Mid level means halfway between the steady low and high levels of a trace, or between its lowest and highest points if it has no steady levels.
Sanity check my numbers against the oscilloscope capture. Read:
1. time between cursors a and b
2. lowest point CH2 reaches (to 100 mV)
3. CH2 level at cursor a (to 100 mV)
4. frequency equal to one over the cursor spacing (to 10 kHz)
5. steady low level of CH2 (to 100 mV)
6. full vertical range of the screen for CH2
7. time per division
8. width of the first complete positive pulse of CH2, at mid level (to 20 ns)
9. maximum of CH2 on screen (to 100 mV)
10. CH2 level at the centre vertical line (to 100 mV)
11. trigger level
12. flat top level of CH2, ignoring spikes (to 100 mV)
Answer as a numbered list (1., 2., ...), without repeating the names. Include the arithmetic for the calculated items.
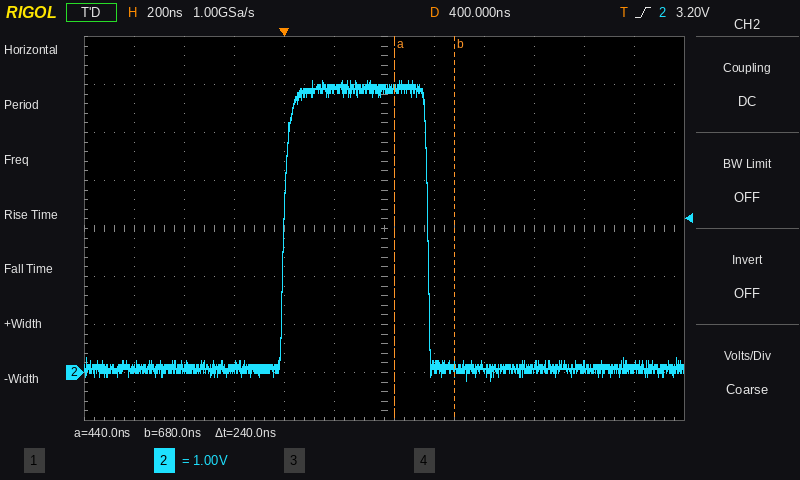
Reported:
1. 240 ns
2. -200 mV
3. 5.9 V
4. 1 / 240 ns ≈ 4.17 MHz
5. 100 mV
6. 8 V
7. 200 ns
8. 580 ns
9. 6.1 V
10. 5.9 V
11. 3.20 V
12. 5.9 V
